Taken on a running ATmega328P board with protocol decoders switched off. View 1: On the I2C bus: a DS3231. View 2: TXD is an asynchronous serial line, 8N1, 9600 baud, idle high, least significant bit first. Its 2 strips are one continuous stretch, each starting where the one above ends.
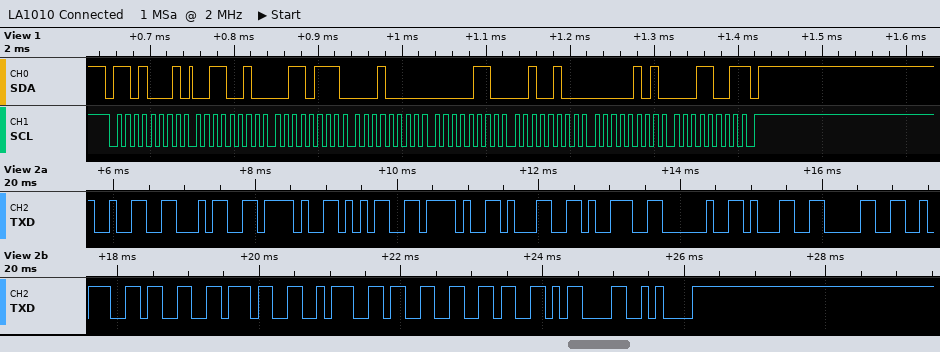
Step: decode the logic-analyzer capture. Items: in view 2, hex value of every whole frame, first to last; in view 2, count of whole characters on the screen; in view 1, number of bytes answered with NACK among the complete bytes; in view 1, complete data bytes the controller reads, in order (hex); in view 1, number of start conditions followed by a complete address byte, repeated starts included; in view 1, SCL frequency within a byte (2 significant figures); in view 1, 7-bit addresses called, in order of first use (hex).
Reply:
32 34 2F 35 2F 31 39 20 31 30 3A 33 37 3A 33 36 0D 0A
18
1
32 37 10 06 24 05 19
1
100 kHz
0x68
